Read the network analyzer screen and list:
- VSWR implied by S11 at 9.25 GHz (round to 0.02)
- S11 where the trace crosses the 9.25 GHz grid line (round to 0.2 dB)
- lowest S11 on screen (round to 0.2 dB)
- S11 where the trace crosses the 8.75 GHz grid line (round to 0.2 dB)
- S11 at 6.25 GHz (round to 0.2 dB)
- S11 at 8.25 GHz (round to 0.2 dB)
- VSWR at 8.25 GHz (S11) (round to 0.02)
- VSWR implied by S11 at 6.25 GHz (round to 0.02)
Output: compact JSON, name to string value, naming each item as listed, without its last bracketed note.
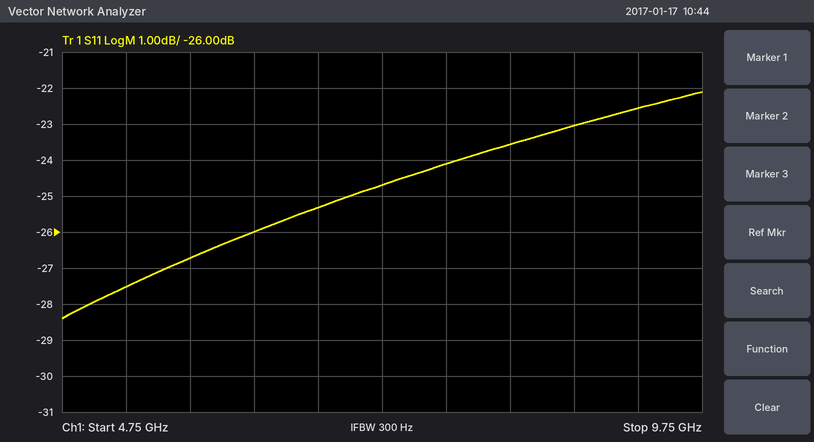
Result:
{"VSWR implied by S11 at 9.25 GHz": "1.16", "S11 where the trace crosses the 9.25 GHz grid line": "-22.6 dB", "lowest S11 on screen": "-28.4 dB", "S11 where the trace crosses the 8.75 GHz grid line": "-23.0 dB", "S11 at 6.25 GHz": "-26.0 dB", "S11 at 8.25 GHz": "-23.6 dB", "VSWR at 8.25 GHz (S11)": "1.14", "VSWR implied by S11 at 6.25 GHz": "1.10"}
